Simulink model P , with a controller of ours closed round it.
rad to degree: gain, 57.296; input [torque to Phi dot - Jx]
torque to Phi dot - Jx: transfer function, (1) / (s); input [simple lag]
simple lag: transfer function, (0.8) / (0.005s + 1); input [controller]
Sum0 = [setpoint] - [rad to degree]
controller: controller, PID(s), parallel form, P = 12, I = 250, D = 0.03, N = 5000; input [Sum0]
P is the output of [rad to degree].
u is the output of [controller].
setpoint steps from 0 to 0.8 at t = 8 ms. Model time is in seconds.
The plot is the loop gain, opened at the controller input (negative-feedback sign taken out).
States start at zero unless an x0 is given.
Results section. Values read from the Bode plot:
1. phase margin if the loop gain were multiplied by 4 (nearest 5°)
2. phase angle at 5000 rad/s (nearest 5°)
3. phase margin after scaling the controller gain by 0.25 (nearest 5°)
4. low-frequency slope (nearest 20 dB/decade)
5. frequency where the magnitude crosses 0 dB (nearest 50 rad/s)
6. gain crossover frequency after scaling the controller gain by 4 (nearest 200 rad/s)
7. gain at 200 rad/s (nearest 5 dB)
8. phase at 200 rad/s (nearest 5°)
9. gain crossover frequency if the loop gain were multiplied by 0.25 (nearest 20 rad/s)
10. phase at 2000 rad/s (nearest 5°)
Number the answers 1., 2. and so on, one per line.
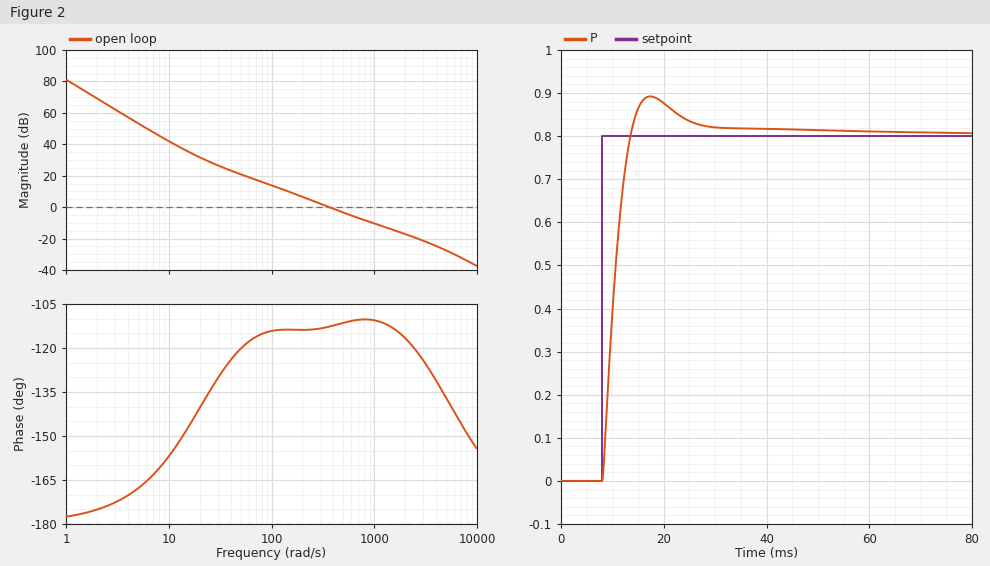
1. 70°
2. -135°
3. 65°
4. -40 dB/decade
5. 350 rad/s
6. 1200 rad/s
7. 5 dB
8. -115°
9. 120 rad/s
10. -115°
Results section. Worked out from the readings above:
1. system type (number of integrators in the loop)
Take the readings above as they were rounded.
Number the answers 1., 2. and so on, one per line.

1. 2
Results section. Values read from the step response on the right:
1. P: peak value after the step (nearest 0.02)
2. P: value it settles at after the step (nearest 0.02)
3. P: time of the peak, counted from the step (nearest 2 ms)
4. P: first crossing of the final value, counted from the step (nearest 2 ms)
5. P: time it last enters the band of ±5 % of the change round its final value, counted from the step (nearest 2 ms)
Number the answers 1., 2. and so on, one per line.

1. 0.90
2. 0.80
3. 10 ms
4. 6 ms
5. 16 ms
